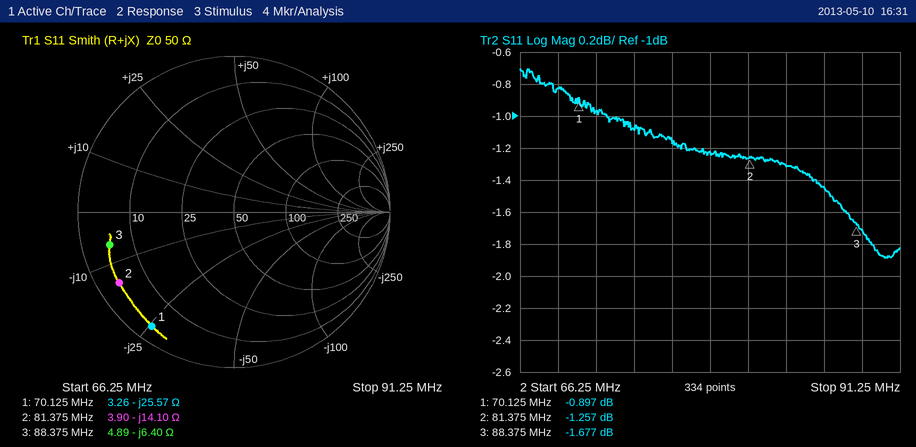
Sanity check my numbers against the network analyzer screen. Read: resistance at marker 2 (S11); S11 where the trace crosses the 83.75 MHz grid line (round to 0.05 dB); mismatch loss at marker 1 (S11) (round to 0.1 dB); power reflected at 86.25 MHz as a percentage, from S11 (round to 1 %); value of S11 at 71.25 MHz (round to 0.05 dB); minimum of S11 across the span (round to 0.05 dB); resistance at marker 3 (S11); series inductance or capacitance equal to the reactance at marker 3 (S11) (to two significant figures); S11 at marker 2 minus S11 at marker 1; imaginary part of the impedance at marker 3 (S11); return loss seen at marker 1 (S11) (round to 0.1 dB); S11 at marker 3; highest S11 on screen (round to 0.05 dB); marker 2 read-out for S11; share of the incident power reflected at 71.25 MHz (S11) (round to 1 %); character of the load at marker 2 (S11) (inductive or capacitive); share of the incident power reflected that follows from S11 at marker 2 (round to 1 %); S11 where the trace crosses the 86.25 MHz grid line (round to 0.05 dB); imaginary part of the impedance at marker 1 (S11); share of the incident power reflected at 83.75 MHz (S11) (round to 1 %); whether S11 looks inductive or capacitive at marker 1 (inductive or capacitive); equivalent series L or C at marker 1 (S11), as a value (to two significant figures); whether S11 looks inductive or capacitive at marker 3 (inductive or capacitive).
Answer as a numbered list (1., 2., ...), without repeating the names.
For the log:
1. 3.90 Ω
2. -1.30 dB
3. 7.3 dB
4. 72 %
5. -0.95 dB
6. -1.90 dB
7. 4.89 Ω
8. 280 pF
9. -0.360 dB
10. -6.40 Ω
11. 0.9 dB
12. -1.677 dB
13. -0.70 dB
14. -1.257 dB
15. 80 %
16. capacitive
17. 75 %
18. -1.45 dB
19. -25.57 Ω
20. 74 %
21. capacitive
22. 89 pF
23. capacitive
